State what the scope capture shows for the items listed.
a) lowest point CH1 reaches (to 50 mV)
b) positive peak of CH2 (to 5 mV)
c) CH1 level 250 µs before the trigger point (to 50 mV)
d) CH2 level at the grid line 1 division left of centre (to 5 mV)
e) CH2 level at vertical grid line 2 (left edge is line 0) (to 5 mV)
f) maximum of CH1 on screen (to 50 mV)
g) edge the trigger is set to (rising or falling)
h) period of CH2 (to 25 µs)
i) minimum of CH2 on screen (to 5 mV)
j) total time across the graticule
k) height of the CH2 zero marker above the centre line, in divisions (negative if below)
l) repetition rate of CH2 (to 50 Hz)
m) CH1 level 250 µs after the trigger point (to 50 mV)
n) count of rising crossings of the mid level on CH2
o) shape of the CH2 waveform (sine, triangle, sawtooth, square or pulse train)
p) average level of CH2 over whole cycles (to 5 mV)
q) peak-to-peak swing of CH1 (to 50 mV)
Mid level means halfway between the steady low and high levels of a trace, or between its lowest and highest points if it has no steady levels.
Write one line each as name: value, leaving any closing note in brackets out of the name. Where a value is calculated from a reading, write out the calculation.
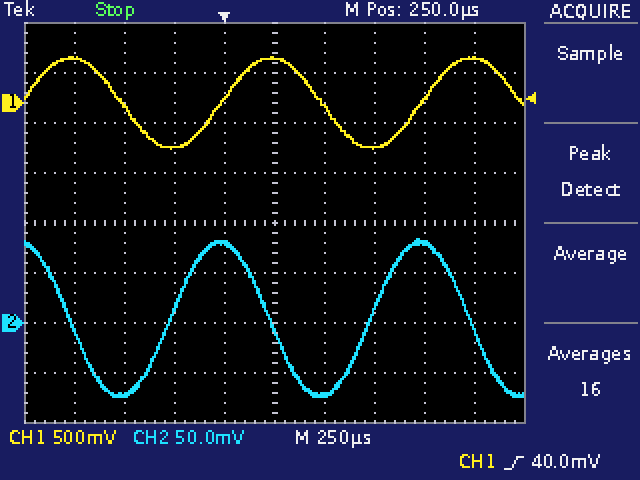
lowest point CH1 reaches: -450 mV
positive peak of CH2: 85 mV
CH1 level 250 µs before the trigger point: -450 mV
CH2 level at the grid line 1 division left of centre: 80 mV
CH2 level at vertical grid line 2 (left edge is line 0): -70 mV
maximum of CH1 on screen: 450 mV
edge the trigger is set to: rising
period of CH2: 1.000 ms
minimum of CH2 on screen: -75 mV
total time across the graticule: 2.5 ms
height of the CH2 zero marker above the centre line, in divisions: -2.0 div
repetition rate of CH2: 1 / 1.000 ms ≈ 1.00 kHz
CH1 level 250 µs after the trigger point: 450 mV
count of rising crossings of the mid level on CH2: 2
shape of the CH2 waveform: sine
average level of CH2 over whole cycles: (85 mV + (-75 mV)) / 2 ≈ 5 mV
peak-to-peak swing of CH1: 450 mV − (-450 mV) = 900 mV
